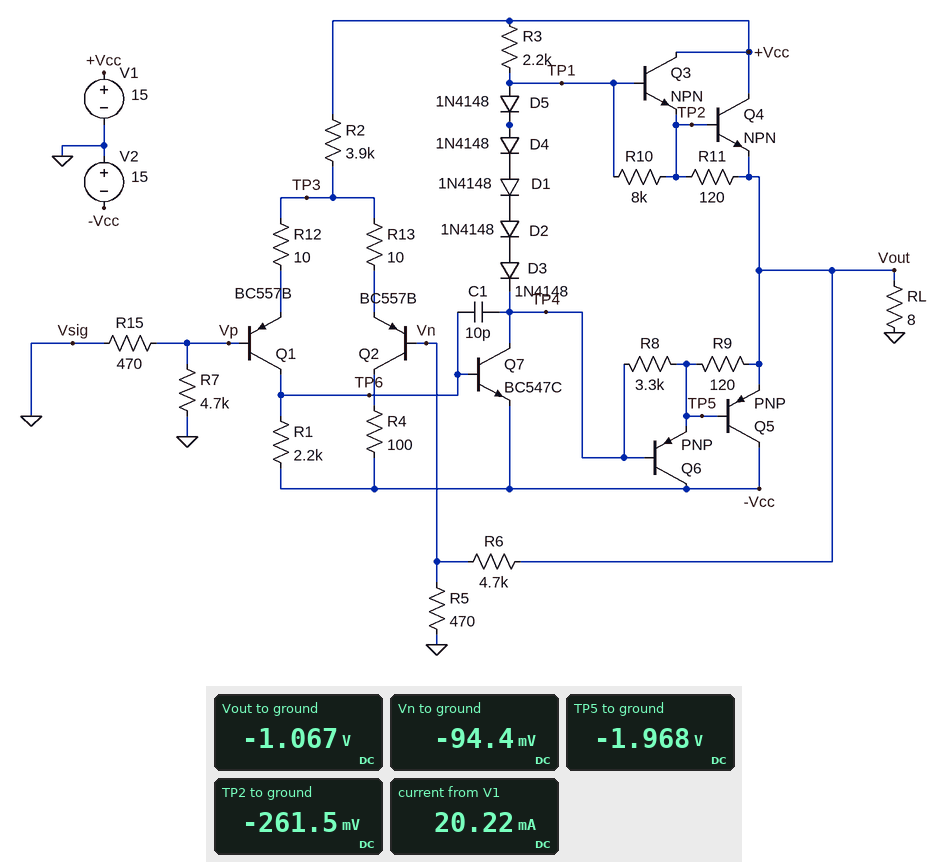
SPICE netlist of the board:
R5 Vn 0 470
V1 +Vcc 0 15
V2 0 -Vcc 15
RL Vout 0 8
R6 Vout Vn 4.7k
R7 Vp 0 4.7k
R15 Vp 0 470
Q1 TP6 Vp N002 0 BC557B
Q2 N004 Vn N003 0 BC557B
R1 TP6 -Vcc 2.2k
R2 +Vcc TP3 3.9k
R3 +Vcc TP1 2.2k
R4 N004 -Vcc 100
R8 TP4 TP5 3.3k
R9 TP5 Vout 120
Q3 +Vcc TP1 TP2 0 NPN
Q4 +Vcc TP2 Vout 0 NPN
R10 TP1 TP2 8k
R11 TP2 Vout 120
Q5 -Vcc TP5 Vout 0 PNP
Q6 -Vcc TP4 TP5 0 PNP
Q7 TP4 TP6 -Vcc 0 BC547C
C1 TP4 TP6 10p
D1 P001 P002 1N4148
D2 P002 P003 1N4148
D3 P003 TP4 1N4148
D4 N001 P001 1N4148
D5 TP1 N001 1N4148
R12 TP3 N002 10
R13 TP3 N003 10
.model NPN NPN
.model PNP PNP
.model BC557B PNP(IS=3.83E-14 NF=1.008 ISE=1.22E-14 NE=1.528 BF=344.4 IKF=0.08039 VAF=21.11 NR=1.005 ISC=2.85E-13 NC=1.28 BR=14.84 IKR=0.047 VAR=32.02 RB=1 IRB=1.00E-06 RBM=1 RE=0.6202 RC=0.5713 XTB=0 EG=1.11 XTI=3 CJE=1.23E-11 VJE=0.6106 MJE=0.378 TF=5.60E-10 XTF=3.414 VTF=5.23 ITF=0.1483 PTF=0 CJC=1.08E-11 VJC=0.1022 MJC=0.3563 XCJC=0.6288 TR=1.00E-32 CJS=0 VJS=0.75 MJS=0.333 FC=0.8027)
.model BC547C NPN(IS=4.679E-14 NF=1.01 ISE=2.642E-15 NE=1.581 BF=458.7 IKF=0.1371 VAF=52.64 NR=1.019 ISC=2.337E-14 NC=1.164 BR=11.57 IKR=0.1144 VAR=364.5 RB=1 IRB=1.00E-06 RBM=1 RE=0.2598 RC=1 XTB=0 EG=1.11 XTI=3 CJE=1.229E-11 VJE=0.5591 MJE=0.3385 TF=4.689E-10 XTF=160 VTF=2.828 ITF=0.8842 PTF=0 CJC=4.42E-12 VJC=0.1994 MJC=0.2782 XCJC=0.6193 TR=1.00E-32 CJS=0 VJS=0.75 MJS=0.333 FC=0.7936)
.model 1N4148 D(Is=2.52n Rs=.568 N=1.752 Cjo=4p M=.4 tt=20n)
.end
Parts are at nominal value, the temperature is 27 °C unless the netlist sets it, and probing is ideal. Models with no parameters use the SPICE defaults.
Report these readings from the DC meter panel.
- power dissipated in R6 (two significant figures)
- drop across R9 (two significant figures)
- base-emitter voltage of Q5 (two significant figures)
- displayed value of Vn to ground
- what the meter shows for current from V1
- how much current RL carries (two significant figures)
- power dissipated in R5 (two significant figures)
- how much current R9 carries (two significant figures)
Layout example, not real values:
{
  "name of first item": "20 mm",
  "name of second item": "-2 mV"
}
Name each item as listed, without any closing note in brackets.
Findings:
{
  "power dissipated in R6": "200 µW",
  "drop across R9": "900 mV",
  "base-emitter voltage of Q5": "-900 mV",
  "displayed value of Vn to ground": "-94.4 mV",
  "what the meter shows for current from V1": "20.22 mA",
  "how much current RL carries": "130 mA",
  "power dissipated in R5": "19 µW",
  "how much current R9 carries": "7.5 mA"
}
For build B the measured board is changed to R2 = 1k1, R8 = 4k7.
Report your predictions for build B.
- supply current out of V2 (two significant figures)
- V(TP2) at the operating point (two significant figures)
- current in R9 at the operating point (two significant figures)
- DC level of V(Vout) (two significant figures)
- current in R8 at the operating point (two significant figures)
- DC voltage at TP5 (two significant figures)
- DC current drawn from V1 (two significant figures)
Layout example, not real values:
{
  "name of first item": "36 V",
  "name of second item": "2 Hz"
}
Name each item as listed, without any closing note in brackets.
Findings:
{
  "supply current out of V2": "360 mA",
  "V(TP2) at the operating point": "-1.9 V",
  "current in R9 at the operating point": "7.7 mA",
  "DC level of V(Vout)": "-2.7 V",
  "current in R8 at the operating point": "180 µA",
  "DC voltage at TP5": "-3.6 V",
  "DC current drawn from V1": "30 mA"
}
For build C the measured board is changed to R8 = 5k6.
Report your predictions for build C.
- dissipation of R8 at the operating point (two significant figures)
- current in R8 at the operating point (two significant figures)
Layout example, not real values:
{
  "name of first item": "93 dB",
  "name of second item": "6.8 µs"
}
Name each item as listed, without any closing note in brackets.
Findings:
{
  "dissipation of R8 at the operating point": "120 µW",
  "current in R8 at the operating point": "150 µA"
}
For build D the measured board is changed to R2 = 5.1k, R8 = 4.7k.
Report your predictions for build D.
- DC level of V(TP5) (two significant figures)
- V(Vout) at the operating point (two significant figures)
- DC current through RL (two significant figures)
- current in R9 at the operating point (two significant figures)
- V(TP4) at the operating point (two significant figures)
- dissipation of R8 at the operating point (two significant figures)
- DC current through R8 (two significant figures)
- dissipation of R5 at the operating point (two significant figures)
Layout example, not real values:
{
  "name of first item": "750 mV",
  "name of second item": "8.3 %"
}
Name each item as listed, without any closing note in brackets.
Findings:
{
  "DC level of V(TP5)": "-1.8 V",
  "V(Vout) at the operating point": "-870 mV",
  "DC current through RL": "110 mA",
  "current in R9 at the operating point": "7.5 mA",
  "V(TP4) at the operating point": "-2.6 V",
  "dissipation of R8 at the operating point": "150 µW",
  "DC current through R8": "180 µA",
  "dissipation of R5 at the operating point": "13 µW"
}
